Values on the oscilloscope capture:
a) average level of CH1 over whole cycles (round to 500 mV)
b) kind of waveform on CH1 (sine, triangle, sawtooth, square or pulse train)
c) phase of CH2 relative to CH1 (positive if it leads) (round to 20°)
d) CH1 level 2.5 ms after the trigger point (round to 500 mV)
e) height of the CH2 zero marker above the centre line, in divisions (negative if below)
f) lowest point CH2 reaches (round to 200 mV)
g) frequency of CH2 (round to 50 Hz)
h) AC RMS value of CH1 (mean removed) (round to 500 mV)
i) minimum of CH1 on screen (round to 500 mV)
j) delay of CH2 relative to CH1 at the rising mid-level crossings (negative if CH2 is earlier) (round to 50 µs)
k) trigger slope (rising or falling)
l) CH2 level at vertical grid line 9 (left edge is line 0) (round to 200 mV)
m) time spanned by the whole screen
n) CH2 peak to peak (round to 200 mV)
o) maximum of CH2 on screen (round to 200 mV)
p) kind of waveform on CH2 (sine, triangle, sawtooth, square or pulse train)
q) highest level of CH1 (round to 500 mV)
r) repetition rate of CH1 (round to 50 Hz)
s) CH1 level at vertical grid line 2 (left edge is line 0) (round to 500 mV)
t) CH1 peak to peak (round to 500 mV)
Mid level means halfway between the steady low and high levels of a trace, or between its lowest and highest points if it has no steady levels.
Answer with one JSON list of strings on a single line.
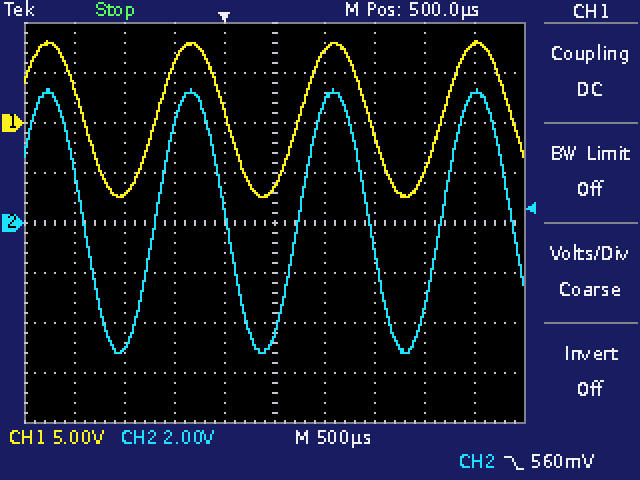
["500 mV", "sine", "0°", "8.0 V", "0.0 div", "-5.2 V", "700 Hz", "5.5 V", "-7.5 V", "0 µs", "falling", "5.2 V", "5 ms", "10.6 V", "5.4 V", "sine", "8.0 V", "700 Hz", "-7.0 V", "15.5 V"]
